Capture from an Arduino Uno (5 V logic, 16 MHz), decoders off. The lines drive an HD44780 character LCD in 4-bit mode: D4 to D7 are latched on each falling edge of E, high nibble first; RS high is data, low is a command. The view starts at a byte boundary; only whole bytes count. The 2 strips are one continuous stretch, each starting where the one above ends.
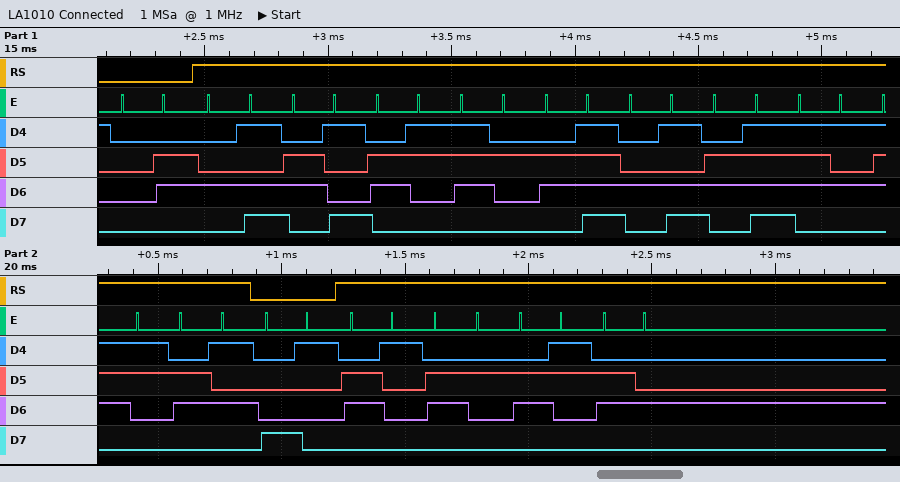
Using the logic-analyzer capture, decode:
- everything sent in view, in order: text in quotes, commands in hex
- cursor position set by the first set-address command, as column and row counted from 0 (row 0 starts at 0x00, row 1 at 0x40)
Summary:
0x06 "MicroMouse" 0x81 "abcd"
column 1, row 0
